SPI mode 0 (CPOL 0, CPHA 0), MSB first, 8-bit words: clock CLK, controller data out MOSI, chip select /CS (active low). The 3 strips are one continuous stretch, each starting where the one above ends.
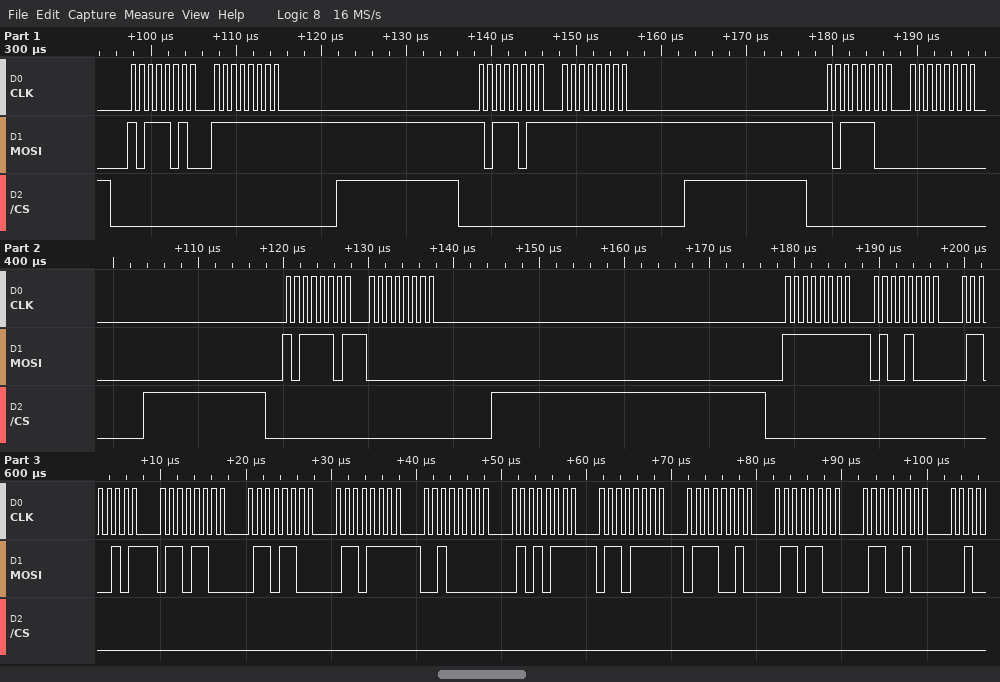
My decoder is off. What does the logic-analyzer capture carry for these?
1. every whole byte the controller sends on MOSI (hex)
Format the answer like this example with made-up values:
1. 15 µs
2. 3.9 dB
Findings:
1. BA FF BB FF BC 00 BD 00 FF 48 65 6C 6C 6F 20 57 6F 72 6C 64
